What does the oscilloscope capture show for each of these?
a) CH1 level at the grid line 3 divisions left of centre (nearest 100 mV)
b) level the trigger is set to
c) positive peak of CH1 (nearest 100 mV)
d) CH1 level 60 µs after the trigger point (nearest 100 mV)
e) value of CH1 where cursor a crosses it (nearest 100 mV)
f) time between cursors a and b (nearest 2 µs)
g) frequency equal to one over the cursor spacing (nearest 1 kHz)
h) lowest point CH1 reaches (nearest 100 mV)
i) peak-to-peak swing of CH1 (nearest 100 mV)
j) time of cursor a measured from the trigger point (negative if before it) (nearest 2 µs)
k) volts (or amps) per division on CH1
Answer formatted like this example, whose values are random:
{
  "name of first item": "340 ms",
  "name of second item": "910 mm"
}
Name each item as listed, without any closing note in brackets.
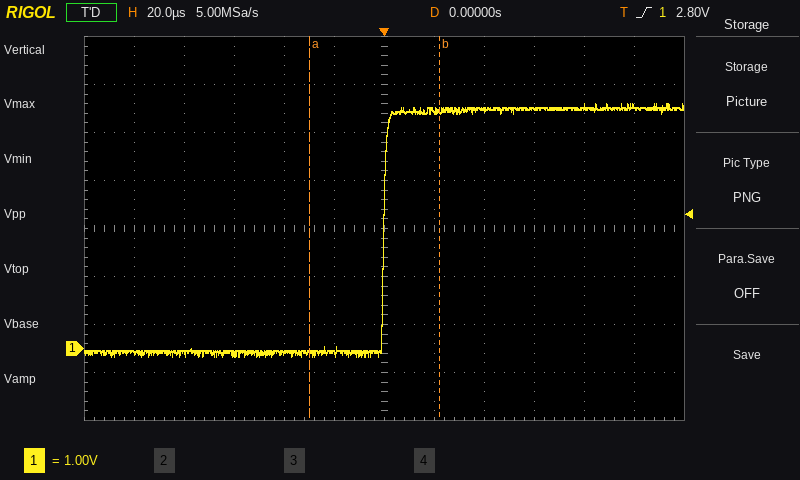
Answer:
{
  "CH1 level at the grid line 3 divisions left of centre": "-100 mV",
  "level the trigger is set to": "2.80 V",
  "positive peak of CH1": "5.1 V",
  "CH1 level 60 µs after the trigger point": "5.0 V",
  "value of CH1 where cursor a crosses it": "-100 mV",
  "time between cursors a and b": "52 µs",
  "frequency equal to one over the cursor spacing": "19 kHz",
  "lowest point CH1 reaches": "-200 mV",
  "peak-to-peak swing of CH1": "5.3 V",
  "time of cursor a measured from the trigger point (negative if before it)": "-30 µs",
  "volts (or amps) per division on CH1": "1 V"
}
